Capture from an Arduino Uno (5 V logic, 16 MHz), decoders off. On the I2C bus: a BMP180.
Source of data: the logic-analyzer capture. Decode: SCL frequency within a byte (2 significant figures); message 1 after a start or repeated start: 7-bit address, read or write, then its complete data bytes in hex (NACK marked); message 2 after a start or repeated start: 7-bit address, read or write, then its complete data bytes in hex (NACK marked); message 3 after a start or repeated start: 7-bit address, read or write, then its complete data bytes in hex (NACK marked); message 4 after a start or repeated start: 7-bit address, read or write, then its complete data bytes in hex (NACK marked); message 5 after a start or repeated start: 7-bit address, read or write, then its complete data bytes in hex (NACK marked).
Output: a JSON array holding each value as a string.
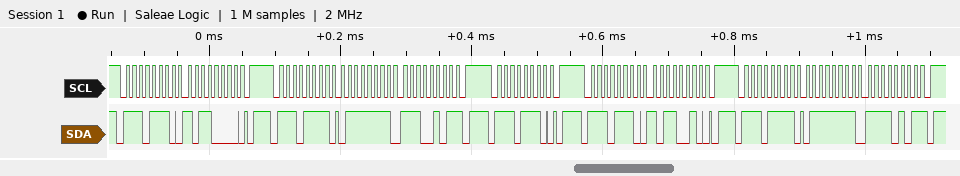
["100 kHz", "0x77 write: B0", "0x77 read: 7F E5 NACK", "0x77 write", "0x77 write: B2", "0x77 read: 7F F5 NACK"]
